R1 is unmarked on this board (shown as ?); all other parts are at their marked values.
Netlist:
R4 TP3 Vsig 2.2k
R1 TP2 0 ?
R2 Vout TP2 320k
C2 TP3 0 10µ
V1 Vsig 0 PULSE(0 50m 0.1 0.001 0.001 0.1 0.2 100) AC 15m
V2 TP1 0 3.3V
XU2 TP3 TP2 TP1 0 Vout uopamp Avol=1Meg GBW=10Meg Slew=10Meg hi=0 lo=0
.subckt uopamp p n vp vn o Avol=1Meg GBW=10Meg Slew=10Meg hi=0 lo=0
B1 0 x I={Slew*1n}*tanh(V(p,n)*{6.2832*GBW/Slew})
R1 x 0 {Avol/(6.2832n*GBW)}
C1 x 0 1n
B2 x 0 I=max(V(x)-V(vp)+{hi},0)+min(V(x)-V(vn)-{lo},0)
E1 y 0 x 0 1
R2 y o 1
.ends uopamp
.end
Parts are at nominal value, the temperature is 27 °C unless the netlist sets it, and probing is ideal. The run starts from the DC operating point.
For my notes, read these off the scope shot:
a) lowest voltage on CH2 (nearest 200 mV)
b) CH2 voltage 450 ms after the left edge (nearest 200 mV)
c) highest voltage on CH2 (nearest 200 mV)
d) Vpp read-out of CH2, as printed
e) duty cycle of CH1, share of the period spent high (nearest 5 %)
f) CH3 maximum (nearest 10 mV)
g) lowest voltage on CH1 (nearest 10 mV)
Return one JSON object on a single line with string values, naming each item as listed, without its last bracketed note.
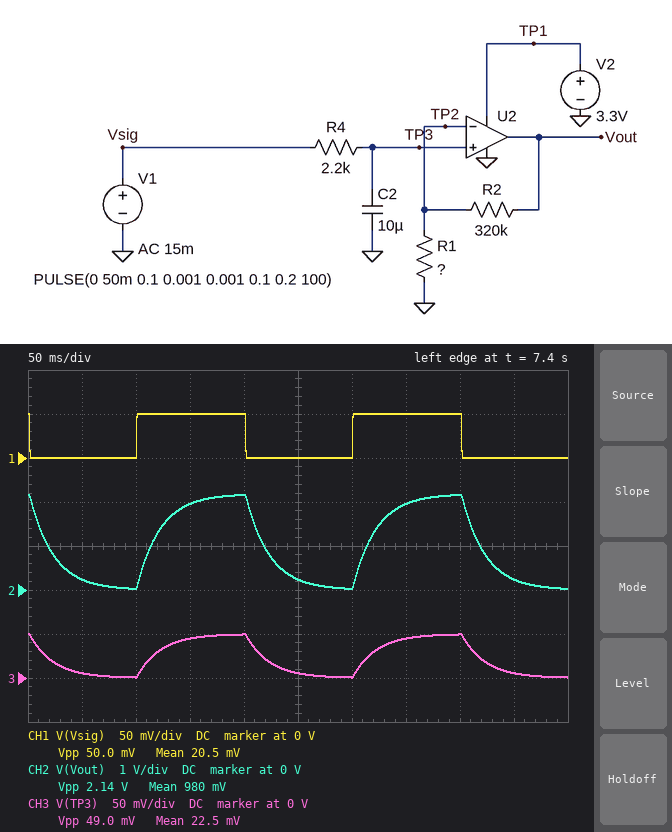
{"lowest voltage on CH2": "0 V", "CH2 voltage 450 ms after the left edge": "200 mV", "highest voltage on CH2": "2.2 V", "Vpp read-out of CH2, as printed": "2.14 V", "duty cycle of CH1, share of the period spent high": "50 %", "CH3 maximum": "50 mV", "lowest voltage on CH1": "0 V"}
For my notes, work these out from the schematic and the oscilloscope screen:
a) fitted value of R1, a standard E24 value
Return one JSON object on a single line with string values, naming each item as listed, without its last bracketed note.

{"fitted value of R1, a standard E24 value": "7.5 kΩ"}
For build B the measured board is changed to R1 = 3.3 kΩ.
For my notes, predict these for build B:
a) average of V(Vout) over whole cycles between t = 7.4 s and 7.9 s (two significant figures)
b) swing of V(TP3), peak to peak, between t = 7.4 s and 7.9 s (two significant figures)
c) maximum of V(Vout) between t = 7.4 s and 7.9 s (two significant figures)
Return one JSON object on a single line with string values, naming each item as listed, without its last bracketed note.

{"average of V(Vout) over whole cycles between t = 7.4 s and 7.9 s": "2.0 V", "swing of V(TP3), peak to peak, between t = 7.4 s and 7.9 s": "49 mV", "maximum of V(Vout) between t = 7.4 s and 7.9 s": "3.3 V"}
